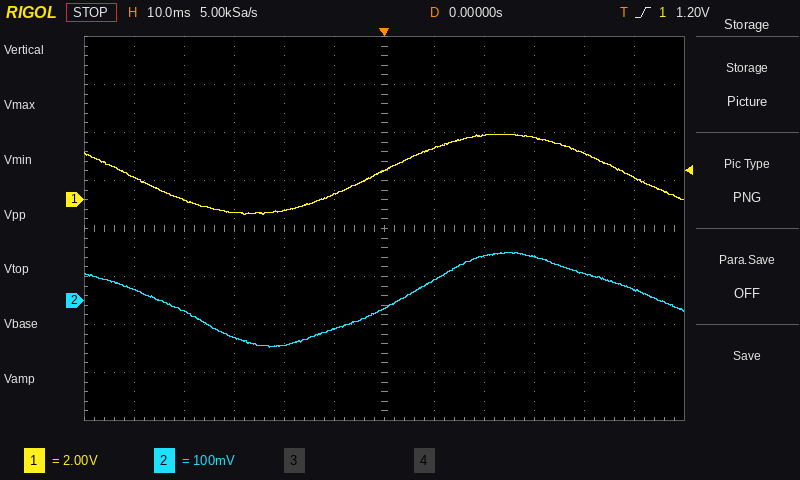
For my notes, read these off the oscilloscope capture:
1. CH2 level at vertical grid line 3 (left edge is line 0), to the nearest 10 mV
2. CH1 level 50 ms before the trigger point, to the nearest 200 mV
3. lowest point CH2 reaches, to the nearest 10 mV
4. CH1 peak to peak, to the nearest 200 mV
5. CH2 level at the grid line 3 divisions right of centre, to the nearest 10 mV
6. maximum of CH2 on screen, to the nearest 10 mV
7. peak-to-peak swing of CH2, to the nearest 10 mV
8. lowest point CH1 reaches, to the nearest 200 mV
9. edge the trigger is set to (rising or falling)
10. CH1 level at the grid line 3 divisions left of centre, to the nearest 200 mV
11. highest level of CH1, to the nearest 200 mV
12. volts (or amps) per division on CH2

-80 mV
1.0 V
-100 mV
3.4 V
90 mV
100 mV
200 mV
-600 mV
rising
-600 mV
2.8 V
100 mV
